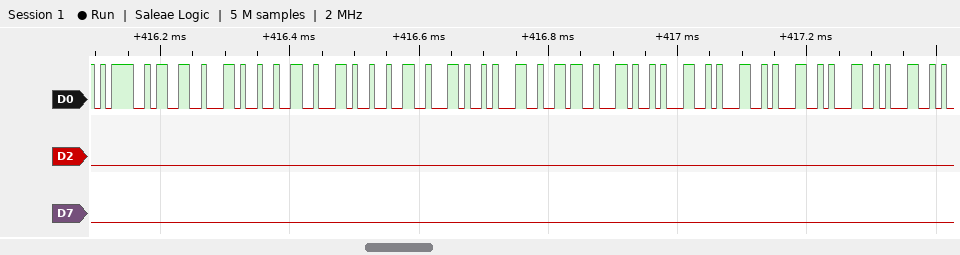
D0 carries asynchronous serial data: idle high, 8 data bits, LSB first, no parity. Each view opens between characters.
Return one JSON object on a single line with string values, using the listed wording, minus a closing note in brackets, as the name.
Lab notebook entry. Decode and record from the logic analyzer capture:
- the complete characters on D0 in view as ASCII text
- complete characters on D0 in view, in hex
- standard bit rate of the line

{"the complete characters on D0 in view as ASCII text": "\"=3,2,2,16,11111\"", "complete characters on D0 in view, in hex": "3D, 33, 2C, 32, 2C, 32, 2C, 31, 36, 2C, 31, 31, 31, 31, 31", "standard bit rate of the line": "115200 baud"}
